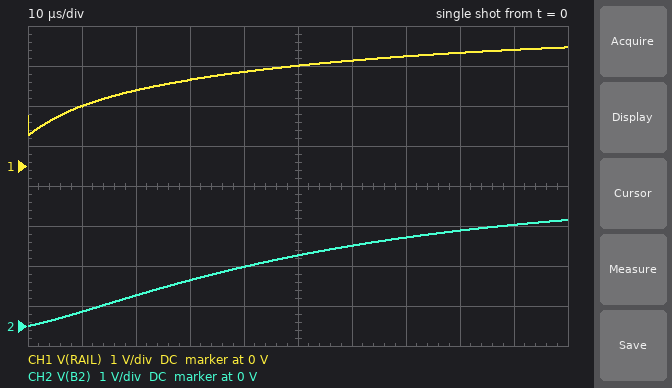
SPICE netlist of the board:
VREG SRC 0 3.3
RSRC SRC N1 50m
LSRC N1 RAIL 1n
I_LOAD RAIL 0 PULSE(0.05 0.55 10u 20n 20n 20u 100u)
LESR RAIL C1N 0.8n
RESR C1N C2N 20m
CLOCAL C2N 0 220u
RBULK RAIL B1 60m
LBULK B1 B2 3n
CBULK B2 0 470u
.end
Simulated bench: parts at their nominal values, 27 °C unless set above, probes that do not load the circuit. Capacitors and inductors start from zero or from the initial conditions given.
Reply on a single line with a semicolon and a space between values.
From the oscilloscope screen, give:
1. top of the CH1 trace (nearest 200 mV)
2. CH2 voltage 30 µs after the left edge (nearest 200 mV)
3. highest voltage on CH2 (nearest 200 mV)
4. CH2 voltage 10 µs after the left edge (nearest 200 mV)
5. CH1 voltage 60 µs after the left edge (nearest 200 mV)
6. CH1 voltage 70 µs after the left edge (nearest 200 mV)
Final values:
3.0 V; 1.2 V; 2.6 V; 400 mV; 2.6 V; 2.8 V
